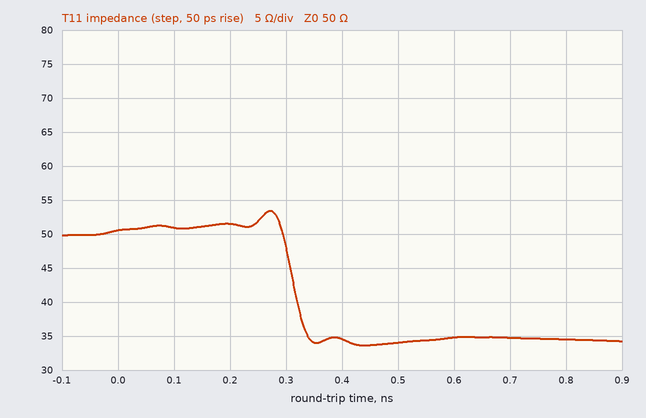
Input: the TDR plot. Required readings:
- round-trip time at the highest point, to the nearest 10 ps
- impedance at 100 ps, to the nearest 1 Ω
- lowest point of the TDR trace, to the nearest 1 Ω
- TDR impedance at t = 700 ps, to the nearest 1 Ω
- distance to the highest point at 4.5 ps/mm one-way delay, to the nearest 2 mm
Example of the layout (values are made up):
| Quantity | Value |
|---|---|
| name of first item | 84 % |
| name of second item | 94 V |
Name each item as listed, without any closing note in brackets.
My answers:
| Quantity | Value |
|---|---|
| round-trip time at the highest point, to the nearest 10 ps | 270 ps |
| impedance at 100 ps, to the nearest 1 Ω | 51 Ω |
| lowest point of the TDR trace, to the nearest 1 Ω | 34 Ω |
| TDR impedance at t = 700 ps, to the nearest 1 Ω | 35 Ω |
| distance to the highest point at 4.5 ps/mm one-way delay, to the nearest 2 mm | 30 mm |
